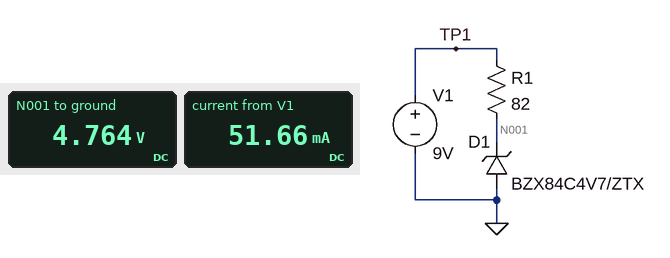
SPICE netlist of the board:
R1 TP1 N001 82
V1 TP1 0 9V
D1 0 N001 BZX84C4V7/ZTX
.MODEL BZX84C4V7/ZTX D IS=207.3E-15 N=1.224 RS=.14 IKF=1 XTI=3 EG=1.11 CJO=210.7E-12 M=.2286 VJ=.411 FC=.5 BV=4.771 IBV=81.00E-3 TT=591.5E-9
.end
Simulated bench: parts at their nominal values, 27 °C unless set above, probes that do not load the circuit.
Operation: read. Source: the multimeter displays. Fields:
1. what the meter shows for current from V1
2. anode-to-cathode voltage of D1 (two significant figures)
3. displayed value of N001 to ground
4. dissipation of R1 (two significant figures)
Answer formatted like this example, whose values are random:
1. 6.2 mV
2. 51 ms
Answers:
1. 51.66 mA
2. -4.8 V
3. 4.764 V
4. 220 mW
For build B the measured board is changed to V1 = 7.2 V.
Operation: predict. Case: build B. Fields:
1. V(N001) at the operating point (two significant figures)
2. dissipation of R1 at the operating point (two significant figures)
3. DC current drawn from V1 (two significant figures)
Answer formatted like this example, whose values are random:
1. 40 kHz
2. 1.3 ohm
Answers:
1. 4.7 V
2. 74 mW
3. 30 mA
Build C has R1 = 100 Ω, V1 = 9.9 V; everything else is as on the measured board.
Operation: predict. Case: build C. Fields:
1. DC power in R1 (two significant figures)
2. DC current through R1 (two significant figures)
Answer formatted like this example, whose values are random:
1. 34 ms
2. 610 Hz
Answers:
1. 260 mW
2. 51 mA
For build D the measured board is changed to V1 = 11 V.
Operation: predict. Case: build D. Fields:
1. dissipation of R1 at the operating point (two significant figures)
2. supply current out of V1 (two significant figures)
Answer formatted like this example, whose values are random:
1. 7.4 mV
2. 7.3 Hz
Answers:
1. 470 mW
2. 76 mA
